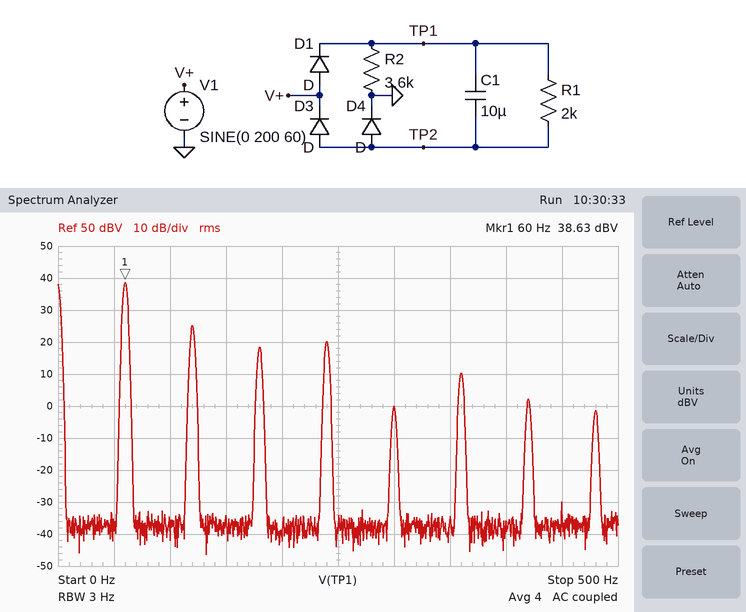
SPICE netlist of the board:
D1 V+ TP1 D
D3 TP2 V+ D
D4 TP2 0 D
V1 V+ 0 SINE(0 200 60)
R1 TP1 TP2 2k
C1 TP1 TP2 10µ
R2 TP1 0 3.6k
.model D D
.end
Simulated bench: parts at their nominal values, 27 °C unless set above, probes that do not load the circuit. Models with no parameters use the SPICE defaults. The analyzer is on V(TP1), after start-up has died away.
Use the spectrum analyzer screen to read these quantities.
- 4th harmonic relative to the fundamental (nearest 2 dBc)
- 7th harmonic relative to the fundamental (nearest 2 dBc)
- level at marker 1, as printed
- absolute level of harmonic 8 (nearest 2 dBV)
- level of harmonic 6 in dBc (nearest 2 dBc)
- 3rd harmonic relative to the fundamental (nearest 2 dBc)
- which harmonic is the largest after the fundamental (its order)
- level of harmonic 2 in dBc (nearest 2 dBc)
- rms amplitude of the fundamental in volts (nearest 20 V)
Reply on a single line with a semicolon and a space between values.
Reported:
-18 dBc; -36 dBc; 38.63 dBV; -2 dBV; -28 dBc; -20 dBc; 2; -14 dBc; 80 V
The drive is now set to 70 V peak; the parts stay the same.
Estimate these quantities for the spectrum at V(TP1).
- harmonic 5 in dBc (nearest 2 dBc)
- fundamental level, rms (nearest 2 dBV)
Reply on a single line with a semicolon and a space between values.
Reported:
-40 dBc; 30 dBV
